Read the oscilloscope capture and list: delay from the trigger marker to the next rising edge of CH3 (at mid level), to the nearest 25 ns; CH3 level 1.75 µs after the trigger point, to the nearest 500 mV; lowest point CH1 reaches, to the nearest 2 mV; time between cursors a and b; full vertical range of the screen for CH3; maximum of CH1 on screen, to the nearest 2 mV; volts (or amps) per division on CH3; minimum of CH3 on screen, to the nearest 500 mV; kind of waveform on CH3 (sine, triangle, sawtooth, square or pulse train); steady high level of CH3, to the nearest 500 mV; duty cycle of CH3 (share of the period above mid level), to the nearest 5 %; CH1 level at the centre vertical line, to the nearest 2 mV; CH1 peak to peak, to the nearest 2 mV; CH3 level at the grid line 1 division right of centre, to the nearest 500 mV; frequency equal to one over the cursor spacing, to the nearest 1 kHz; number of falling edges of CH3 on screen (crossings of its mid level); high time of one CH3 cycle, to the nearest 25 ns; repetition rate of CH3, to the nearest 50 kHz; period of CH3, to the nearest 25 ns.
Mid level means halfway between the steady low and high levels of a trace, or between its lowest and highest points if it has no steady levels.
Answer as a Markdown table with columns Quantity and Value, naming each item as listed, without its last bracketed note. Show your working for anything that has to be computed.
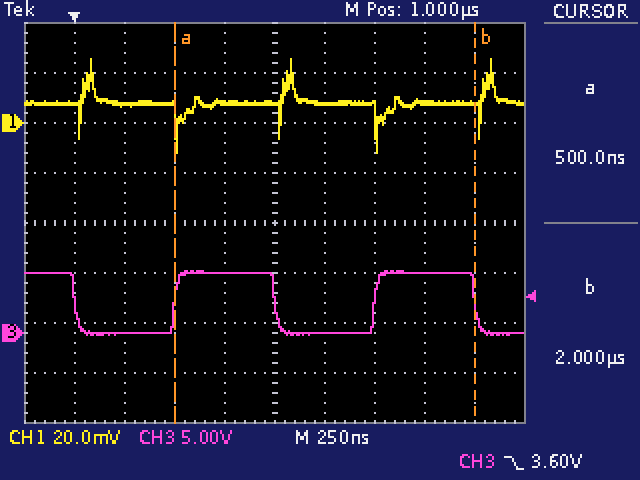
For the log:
| Quantity | Value |
|---|---|
| delay from the trigger marker to the next rising edge of CH3 (at mid level), to the nearest 25 ns | 500 ns |
| CH3 level 1.75 µs after the trigger point, to the nearest 500 mV | 6.0 V |
| lowest point CH1 reaches, to the nearest 2 mV | -12 mV |
| time between cursors a and b | 2 µs − (500 ns) = 1.500 µs |
| full vertical range of the screen for CH3 | 40 V |
| maximum of CH1 on screen, to the nearest 2 mV | 26 mV |
| volts (or amps) per division on CH3 | 5 V |
| minimum of CH3 on screen, to the nearest 500 mV | 0.0 V |
| kind of waveform on CH3 | square |
| steady high level of CH3, to the nearest 500 mV | 6.0 V |
| duty cycle of CH3 (share of the period above mid level), to the nearest 5 % | 500 ns / 1.000 µs ≈ 50 % |
| CH1 level at the centre vertical line, to the nearest 2 mV | 8 mV |
| CH1 peak to peak, to the nearest 2 mV | 26 mV − (-12 mV) = 38 mV |
| CH3 level at the grid line 1 division right of centre, to the nearest 500 mV | 0.0 V |
| frequency equal to one over the cursor spacing, to the nearest 1 kHz | 1 / 1.500 µs ≈ 667 kHz |
| number of falling edges of CH3 on screen | 3 |
| high time of one CH3 cycle, to the nearest 25 ns | 500 ns |
| repetition rate of CH3, to the nearest 50 kHz | 1 / 1.000 µs ≈ 1.00 MHz |
| period of CH3, to the nearest 25 ns | 1.000 µs |
